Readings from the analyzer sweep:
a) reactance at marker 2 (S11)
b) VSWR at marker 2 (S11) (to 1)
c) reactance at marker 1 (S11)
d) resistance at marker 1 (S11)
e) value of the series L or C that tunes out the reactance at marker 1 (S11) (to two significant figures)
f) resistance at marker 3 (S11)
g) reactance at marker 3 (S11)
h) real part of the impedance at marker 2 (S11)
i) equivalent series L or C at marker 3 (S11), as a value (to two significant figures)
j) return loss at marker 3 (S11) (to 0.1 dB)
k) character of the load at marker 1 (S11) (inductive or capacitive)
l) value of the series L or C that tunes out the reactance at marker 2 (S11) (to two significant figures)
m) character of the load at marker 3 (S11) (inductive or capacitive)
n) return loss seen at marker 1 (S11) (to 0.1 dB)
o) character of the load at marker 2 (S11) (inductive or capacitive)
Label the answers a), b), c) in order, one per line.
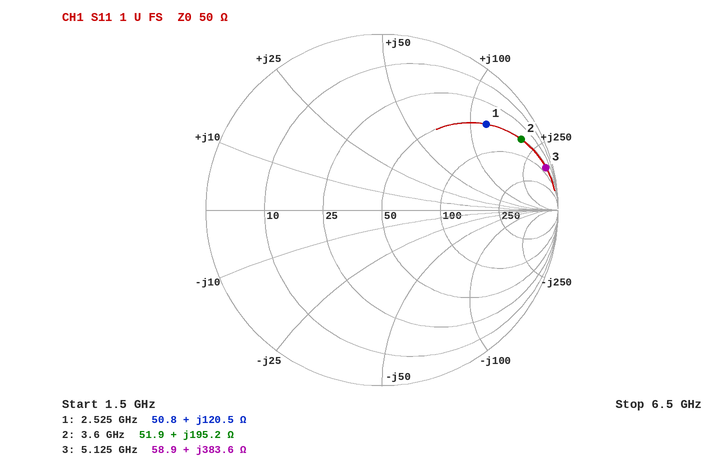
a) +195.2 Ω
b) 17
c) +120.5 Ω
d) 50.8 Ω
e) 520 fF
f) 58.9 Ω
g) +383.6 Ω
h) 51.9 Ω
i) 12 nH
j) 0.3 dB
k) inductive
l) 230 fF
m) inductive
n) 2.3 dB
o) inductive
